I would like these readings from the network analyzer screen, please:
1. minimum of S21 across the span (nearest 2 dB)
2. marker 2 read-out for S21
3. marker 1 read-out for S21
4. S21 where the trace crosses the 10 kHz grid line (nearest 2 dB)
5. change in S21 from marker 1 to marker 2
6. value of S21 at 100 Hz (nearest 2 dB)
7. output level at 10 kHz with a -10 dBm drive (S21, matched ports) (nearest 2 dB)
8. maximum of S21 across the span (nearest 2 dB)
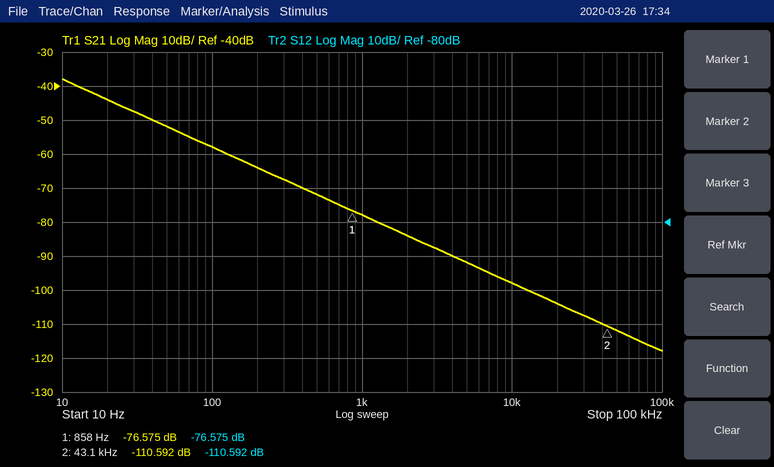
-118 dB
-110.592 dB
-76.575 dB
-98 dB
-34.017 dB
-58 dB
-108 dBm
-38 dB
